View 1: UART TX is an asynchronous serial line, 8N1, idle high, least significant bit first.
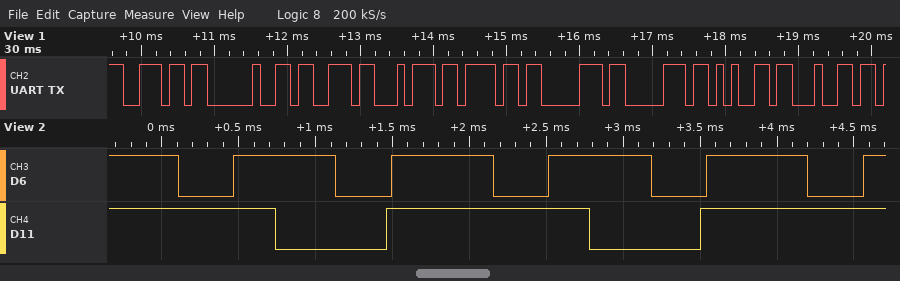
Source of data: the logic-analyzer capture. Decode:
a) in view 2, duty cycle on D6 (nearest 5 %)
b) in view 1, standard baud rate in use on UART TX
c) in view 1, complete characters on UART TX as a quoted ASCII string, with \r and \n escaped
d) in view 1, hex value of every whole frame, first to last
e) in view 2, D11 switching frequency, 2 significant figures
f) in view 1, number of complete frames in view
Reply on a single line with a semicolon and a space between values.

65 %; 9600 baud; "n stopped"; 6E 20 73 74 6F 70 70 65 64; 490 Hz; 9
